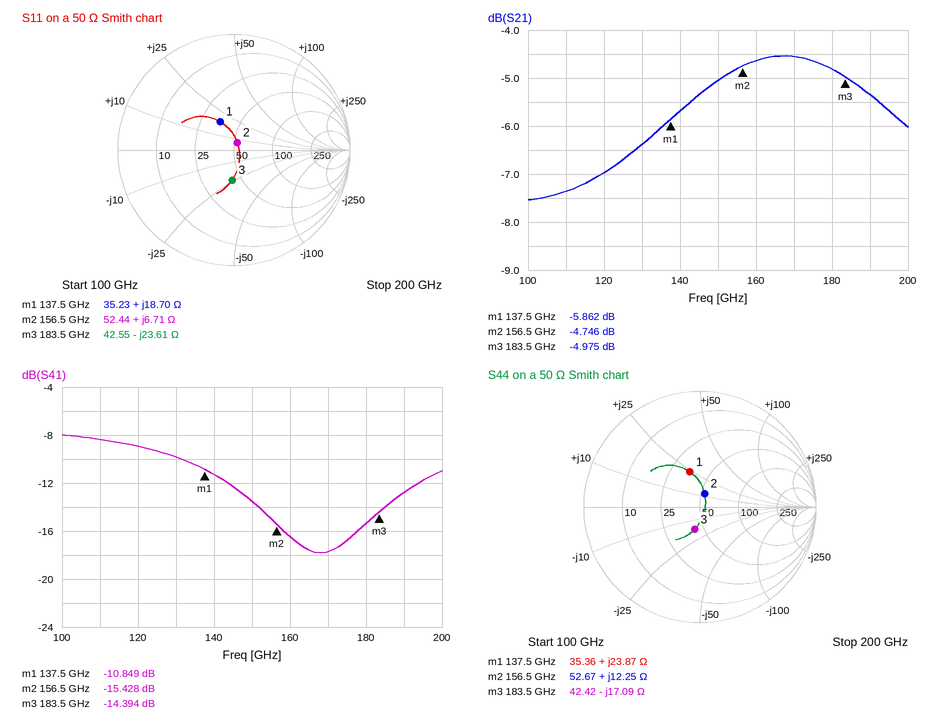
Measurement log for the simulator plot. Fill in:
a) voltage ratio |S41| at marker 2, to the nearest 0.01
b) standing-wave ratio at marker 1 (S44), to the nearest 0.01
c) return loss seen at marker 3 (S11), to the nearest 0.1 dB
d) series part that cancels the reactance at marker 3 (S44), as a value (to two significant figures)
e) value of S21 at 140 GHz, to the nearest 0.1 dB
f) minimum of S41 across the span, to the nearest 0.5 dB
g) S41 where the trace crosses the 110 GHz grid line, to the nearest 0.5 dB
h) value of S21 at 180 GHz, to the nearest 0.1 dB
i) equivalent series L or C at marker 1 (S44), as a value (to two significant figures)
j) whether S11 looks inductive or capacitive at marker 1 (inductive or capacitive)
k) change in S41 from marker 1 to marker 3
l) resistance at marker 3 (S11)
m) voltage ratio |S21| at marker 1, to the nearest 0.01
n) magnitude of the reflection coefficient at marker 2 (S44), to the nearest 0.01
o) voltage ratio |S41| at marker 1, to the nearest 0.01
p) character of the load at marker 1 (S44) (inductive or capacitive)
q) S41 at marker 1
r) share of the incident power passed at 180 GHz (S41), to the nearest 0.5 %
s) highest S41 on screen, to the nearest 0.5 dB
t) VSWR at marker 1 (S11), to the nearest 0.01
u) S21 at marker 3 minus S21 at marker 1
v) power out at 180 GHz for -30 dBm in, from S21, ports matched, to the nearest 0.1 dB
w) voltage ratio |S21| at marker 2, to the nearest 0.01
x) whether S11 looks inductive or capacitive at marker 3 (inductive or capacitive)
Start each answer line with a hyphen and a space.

- 0.17
- 1.92
- 11.7 dB
- 15 pH
- -5.7 dB
- -18.0 dB
- -8.5 dB
- -4.8 dB
- 28 pH
- inductive
- -3.545 dB
- 42.55 Ω
- 0.51
- 0.12
- 0.29
- inductive
- -10.849 dB
- 3.0 %
- -8.0 dB
- 1.75
- 0.887 dB
- -34.8 dBm
- 0.58
- capacitive
